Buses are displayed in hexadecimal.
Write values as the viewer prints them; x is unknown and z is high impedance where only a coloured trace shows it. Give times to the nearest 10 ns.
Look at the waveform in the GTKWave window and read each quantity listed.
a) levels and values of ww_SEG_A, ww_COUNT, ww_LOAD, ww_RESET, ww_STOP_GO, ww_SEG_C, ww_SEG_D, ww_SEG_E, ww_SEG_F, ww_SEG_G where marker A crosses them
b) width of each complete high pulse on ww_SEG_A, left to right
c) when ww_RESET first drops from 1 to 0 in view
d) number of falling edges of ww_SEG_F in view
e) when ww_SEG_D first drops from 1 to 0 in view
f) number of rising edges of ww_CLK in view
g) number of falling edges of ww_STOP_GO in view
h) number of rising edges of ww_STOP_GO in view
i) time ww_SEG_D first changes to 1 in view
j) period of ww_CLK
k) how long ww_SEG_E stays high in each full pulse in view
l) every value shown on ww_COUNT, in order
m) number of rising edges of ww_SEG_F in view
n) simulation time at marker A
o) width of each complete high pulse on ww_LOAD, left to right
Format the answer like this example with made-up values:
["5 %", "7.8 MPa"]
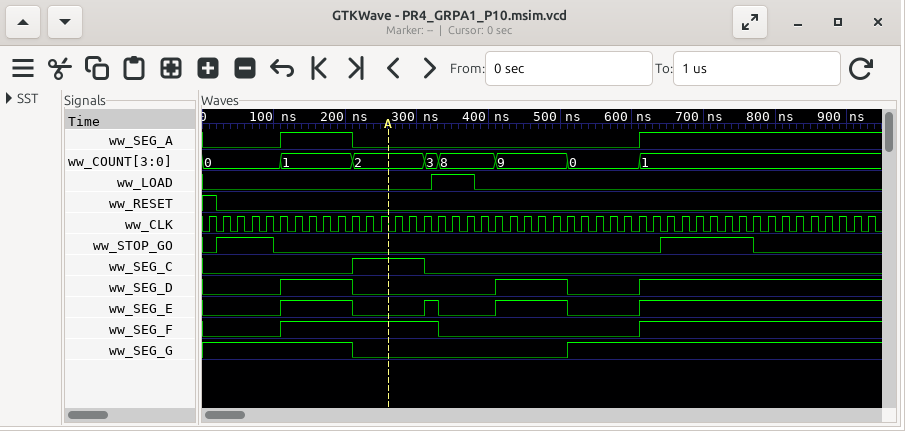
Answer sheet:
["ww_SEG_A=0, ww_COUNT=2, ww_LOAD=0, ww_RESET=0, ww_STOP_GO=0, ww_SEG_C=1, ww_SEG_D=0, ww_SEG_E=0, ww_SEG_F=1, ww_SEG_G=0", "100 ns", "20 ns", "1", "210 ns", "47", "2", "2", "110 ns", "20 ns", "100 ns, 20 ns, 100 ns", "0, 1, 2, 3, 8, 9, 0, 1", "2", "260 ns", "60 ns"]
